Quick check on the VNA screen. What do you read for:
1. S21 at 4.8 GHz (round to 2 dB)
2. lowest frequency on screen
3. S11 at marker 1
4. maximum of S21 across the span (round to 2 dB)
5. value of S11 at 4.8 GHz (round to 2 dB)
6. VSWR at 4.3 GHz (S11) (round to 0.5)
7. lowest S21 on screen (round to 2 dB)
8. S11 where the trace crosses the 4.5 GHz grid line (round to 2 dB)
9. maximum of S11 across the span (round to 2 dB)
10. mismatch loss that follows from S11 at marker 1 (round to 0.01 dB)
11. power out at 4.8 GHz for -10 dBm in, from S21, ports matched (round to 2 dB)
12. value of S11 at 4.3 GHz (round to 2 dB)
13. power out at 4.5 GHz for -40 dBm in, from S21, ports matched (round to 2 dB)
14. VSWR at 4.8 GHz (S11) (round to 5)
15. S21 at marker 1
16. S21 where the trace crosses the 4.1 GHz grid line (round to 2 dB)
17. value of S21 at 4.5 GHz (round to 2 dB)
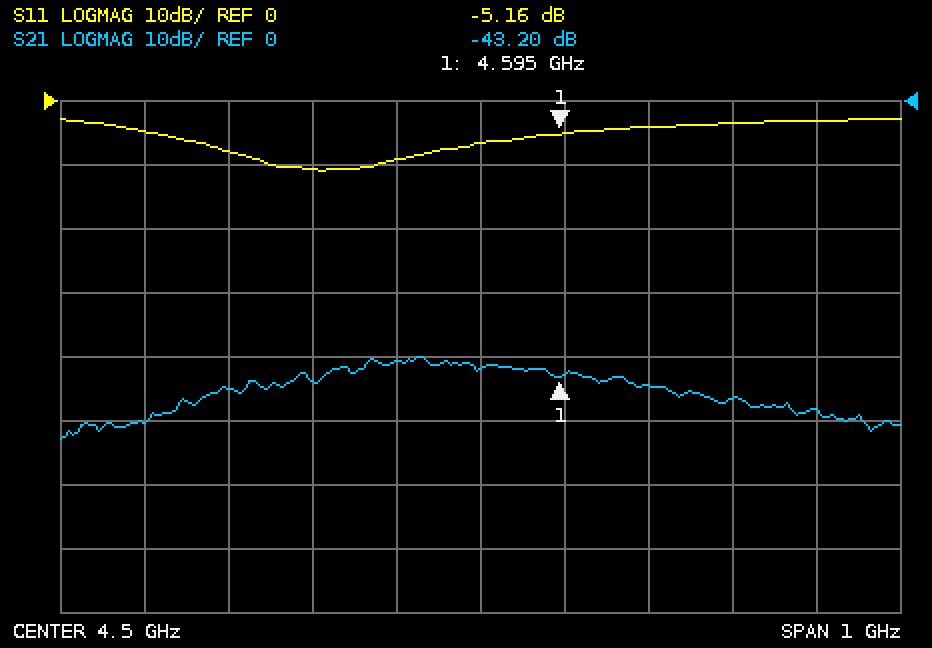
-46 dB
4 GHz
-5.16 dB
-40 dB
-4 dB
2.0
-52 dB
-6 dB
-2 dB
1.58 dB
-56 dBm
-10 dB
-82 dBm
5
-43.20 dB
-50 dB
-42 dB
